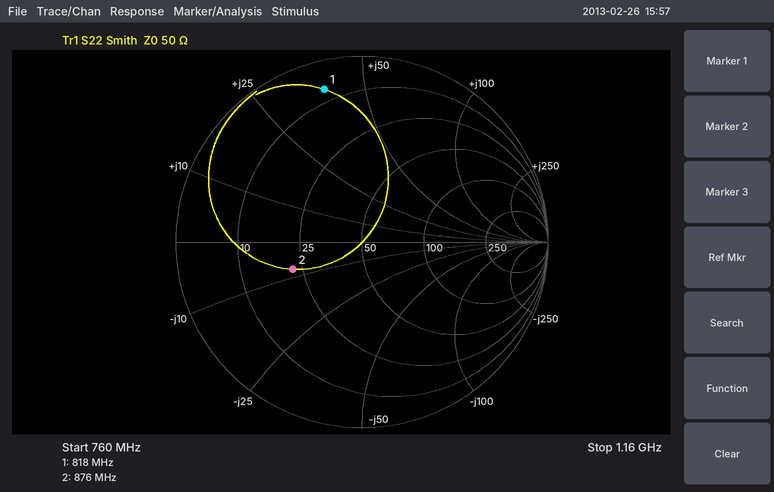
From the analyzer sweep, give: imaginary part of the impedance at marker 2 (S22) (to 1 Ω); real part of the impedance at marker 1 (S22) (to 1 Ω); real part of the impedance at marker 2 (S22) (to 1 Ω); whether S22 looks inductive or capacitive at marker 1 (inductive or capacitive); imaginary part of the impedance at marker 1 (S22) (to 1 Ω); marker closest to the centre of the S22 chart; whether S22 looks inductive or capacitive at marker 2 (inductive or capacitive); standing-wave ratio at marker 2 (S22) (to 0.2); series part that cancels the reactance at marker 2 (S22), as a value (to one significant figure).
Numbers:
-8 Ω
7 Ω
22 Ω
inductive
+39 Ω
marker 2
capacitive
2.4
1 nH
